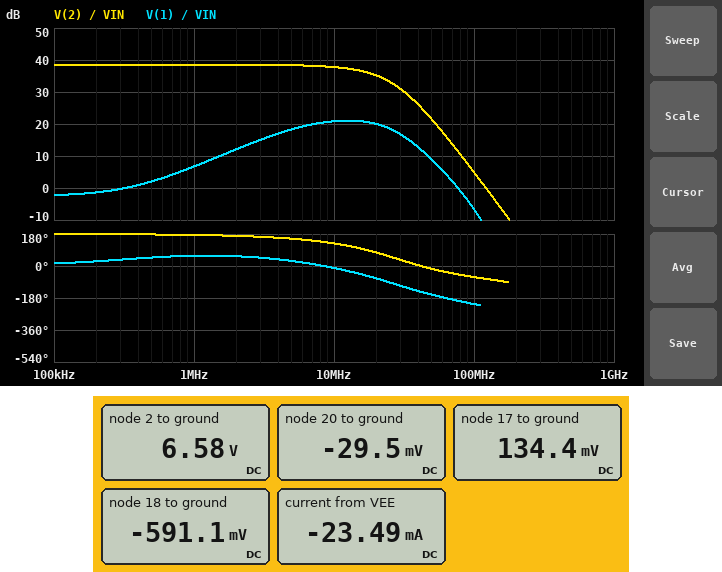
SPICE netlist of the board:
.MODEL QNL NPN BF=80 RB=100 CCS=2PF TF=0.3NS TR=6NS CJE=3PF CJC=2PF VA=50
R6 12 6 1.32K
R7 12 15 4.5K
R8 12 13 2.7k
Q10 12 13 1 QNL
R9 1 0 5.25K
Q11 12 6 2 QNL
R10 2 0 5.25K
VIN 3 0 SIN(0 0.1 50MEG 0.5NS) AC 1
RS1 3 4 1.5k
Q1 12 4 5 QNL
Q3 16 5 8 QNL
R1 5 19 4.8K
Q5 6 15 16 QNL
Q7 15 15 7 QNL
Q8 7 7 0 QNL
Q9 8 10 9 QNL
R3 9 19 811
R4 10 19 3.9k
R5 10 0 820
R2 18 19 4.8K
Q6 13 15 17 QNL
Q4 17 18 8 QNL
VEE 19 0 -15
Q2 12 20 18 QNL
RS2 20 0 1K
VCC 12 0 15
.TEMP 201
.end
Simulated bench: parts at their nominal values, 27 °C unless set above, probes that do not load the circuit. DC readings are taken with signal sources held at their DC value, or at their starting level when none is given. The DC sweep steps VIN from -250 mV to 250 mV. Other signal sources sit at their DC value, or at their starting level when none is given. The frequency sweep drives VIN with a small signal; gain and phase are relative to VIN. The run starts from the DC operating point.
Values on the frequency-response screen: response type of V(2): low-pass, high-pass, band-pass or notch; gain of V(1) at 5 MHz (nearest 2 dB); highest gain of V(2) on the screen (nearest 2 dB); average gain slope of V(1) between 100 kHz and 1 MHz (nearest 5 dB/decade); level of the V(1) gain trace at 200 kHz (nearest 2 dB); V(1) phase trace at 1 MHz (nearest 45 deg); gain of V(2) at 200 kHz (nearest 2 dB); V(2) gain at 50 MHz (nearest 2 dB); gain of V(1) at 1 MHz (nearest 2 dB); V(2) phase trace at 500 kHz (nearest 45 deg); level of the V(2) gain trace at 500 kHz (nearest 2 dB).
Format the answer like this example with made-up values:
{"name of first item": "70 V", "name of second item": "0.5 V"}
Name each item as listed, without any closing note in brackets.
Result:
{"response type of V(2): low-pass, high-pass, band-pass or notch": "low-pass", "gain of V(1) at 5 MHz": "18 dB", "highest gain of V(2) on the screen": "38 dB", "average gain slope of V(1) between 100 kHz and 1 MHz": "10 dB/decade", "level of the V(1) gain trace at 200 kHz": "-2 dB", "V(1) phase trace at 1 MHz": "45 deg", "gain of V(2) at 200 kHz": "38 dB", "V(2) gain at 50 MHz": "22 dB", "gain of V(1) at 1 MHz": "6 dB", "V(2) phase trace at 500 kHz": "180 deg", "level of the V(2) gain trace at 500 kHz": "38 dB"}
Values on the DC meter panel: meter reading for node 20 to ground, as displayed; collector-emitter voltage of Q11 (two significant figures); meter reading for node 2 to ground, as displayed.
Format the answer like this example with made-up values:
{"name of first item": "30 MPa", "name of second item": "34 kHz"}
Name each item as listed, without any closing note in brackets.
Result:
{"meter reading for node 20 to ground, as displayed": "-29.5 mV", "collector-emitter voltage of Q11": "8.4 V", "meter reading for node 2 to ground, as displayed": "6.58 V"}
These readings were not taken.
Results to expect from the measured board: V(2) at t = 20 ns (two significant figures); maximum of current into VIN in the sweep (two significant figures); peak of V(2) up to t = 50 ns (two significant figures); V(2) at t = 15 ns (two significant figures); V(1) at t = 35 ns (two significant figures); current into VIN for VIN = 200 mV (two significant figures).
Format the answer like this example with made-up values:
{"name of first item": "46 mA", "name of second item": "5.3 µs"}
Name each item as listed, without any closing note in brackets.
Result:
{"V(2) at t = 20 ns": "5.1 V", "maximum of current into VIN in the sweep": "-28 µA", "peak of V(2) up to t = 50 ns": "7.8 V", "V(2) at t = 15 ns": "4.1 V", "V(1) at t = 35 ns": "210 mV", "current into VIN for VIN = 200 mV": "-31 µA"}
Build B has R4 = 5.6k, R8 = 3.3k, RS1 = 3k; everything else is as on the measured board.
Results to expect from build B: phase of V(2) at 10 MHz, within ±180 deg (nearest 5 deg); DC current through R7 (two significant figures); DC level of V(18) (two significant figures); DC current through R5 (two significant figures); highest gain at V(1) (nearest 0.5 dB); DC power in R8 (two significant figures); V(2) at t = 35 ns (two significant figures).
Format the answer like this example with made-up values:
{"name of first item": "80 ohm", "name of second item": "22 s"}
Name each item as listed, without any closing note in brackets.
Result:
{"phase of V(2) at 10 MHz, within ±180 deg": "155 deg", "DC current through R7": "3.4 mA", "DC level of V(18)": "-600 mV", "DC current through R5": "2.5 mA", "highest gain at V(1)": "1.0 dB", "DC power in R8": "78 mW", "V(2) at t = 35 ns": "5.6 V"}
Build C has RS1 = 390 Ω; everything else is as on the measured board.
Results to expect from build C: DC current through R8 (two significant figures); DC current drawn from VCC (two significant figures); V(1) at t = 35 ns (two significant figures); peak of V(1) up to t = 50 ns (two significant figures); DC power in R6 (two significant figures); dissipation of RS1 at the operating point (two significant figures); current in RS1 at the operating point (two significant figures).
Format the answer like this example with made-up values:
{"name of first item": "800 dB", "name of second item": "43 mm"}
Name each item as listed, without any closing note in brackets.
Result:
{"DC current through R8": "5.3 mA", "DC current drawn from VCC": "23 mA", "V(1) at t = 35 ns": "950 mV", "peak of V(1) up to t = 50 ns": "2.9 V", "DC power in R6": "87 mW", "dissipation of RS1 at the operating point": "340 nW", "current in RS1 at the operating point": "30 µA"}
